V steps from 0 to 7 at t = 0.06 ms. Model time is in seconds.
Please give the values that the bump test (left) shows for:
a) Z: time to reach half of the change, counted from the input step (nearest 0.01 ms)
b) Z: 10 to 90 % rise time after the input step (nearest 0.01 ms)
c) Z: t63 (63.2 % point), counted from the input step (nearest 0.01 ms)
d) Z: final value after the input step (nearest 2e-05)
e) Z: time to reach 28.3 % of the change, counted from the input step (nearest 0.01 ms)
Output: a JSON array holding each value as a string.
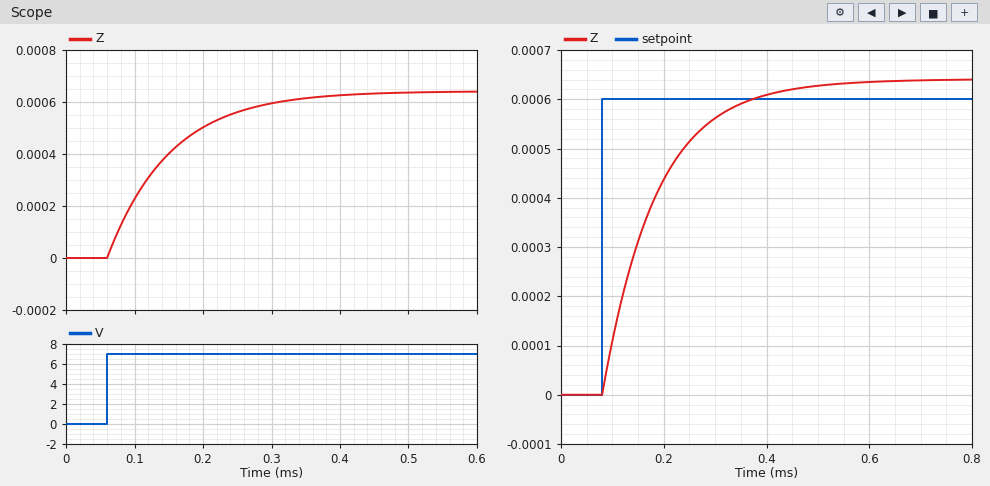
["0.06 ms", "0.20 ms", "0.09 ms", "0.00064", "0.03 ms"]
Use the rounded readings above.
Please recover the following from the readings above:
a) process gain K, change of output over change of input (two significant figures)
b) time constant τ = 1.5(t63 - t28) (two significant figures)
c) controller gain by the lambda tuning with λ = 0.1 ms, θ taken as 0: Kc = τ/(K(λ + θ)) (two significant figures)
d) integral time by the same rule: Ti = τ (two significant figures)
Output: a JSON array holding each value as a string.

["0.000091", "0.090 ms", "9900", "0.090 ms"]
